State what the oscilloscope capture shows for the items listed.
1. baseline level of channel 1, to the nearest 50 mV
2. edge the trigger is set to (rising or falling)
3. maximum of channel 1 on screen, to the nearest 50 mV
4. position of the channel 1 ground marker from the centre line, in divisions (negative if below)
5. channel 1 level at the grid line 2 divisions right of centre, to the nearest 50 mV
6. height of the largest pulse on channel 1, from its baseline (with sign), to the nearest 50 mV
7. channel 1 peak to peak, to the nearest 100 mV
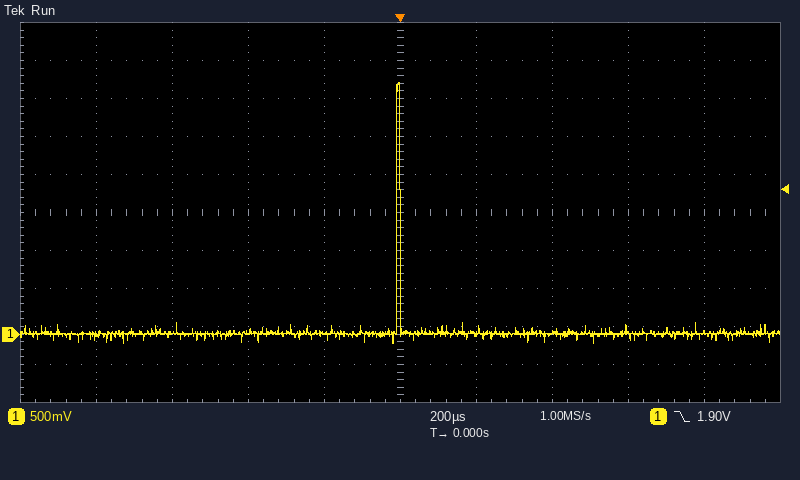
0 mV
falling
3.30 V
-3.2 div
0 mV
+3.30 V
3.40 V
